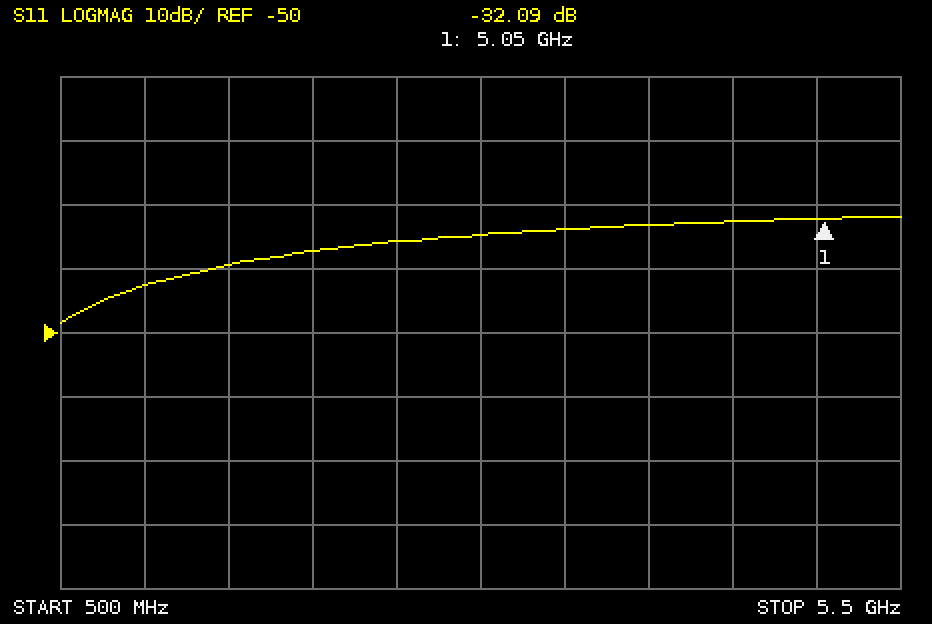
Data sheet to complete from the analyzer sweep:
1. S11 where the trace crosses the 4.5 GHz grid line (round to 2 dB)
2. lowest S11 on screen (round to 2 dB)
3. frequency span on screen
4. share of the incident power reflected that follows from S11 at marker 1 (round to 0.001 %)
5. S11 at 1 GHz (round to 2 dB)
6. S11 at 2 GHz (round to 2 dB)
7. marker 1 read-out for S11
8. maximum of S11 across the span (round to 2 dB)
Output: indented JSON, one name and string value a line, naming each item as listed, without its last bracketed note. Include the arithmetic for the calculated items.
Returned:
{
  "S11 where the trace crosses the 4.5 GHz grid line": "-32 dB",
  "lowest S11 on screen": "-48 dB",
  "frequency span on screen": "5 GHz",
  "share of the incident power reflected that follows from S11 at marker 1": "10^(-32.09/10) ≈ 0.062 %",
  "S11 at 1 GHz": "-42 dB",
  "S11 at 2 GHz": "-38 dB",
  "marker 1 read-out for S11": "-32.09 dB",
  "maximum of S11 across the span": "-32 dB"
}
